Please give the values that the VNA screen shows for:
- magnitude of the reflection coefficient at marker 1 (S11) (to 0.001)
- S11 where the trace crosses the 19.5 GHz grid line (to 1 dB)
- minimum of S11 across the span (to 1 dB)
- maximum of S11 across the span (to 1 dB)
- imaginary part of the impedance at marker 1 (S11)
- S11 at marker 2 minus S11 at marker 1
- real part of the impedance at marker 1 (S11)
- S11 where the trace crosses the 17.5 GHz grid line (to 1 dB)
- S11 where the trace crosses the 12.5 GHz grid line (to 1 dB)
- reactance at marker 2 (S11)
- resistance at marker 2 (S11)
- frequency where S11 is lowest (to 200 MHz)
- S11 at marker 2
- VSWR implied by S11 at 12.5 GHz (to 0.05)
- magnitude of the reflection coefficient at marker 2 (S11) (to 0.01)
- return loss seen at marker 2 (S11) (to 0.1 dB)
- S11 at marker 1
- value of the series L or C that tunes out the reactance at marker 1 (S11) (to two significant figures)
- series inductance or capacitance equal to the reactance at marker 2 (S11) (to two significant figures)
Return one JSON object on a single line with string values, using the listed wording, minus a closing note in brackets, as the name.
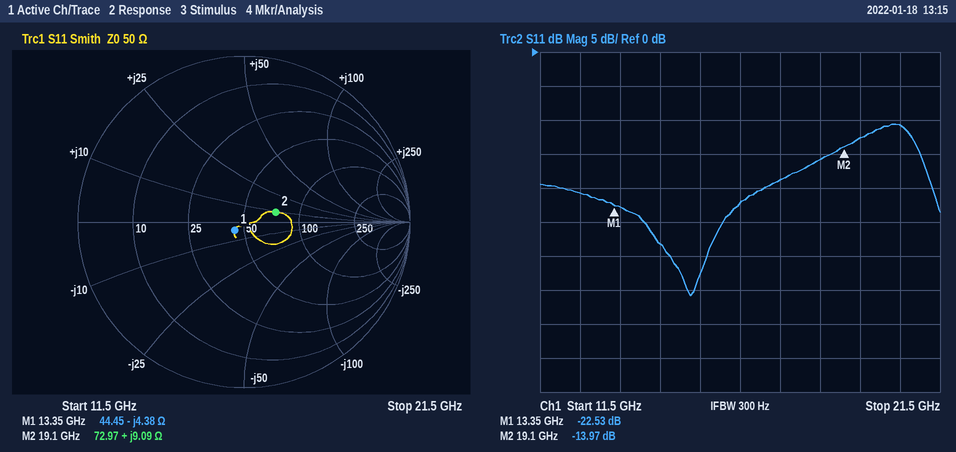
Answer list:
{"magnitude of the reflection coefficient at marker 1 (S11)": "0.075", "S11 where the trace crosses the 19.5 GHz grid line": "-13 dB", "minimum of S11 across the span": "-36 dB", "maximum of S11 across the span": "-11 dB", "imaginary part of the impedance at marker 1": "-4.38 Ω", "S11 at marker 2 minus S11 at marker 1": "8.56 dB", "real part of the impedance at marker 1": "44.45 Ω", "S11 where the trace crosses the 17.5 GHz grid line": "-19 dB", "S11 where the trace crosses the 12.5 GHz grid line": "-21 dB", "reactance at marker 2": "+9.09 Ω", "resistance at marker 2": "72.97 Ω", "frequency where S11 is lowest": "15.2 GHz", "S11 at marker 2": "-13.97 dB", "VSWR implied by S11 at 12.5 GHz": "1.20", "magnitude of the reflection coefficient at marker 2 (S11)": "0.20", "return loss seen at marker 2 (S11)": "14.0 dB", "S11 at marker 1": "-22.53 dB", "value of the series L or C that tunes out the reactance at marker 1 (S11)": "52 pH", "series inductance or capacitance equal to the reactance at marker 2 (S11)": "76 pH"}
